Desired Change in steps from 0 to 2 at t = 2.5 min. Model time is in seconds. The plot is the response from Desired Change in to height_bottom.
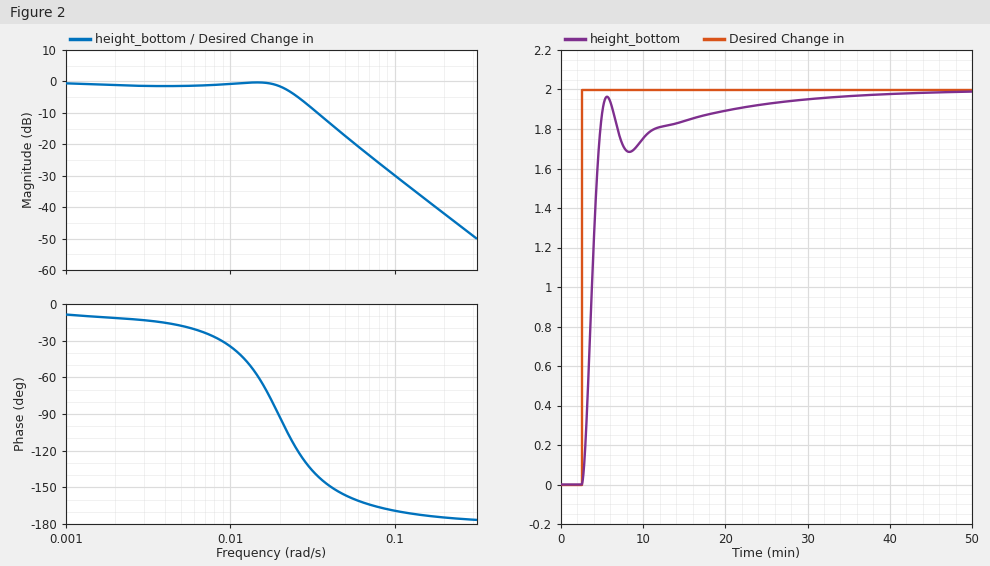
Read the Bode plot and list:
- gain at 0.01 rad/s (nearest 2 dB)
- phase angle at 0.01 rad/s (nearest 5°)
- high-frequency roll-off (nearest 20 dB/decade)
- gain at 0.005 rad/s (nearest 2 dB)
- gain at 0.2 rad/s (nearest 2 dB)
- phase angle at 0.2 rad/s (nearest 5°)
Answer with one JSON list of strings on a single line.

["0 dB", "-35°", "-40 dB/decade", "-2 dB", "-42 dB", "-175°"]
